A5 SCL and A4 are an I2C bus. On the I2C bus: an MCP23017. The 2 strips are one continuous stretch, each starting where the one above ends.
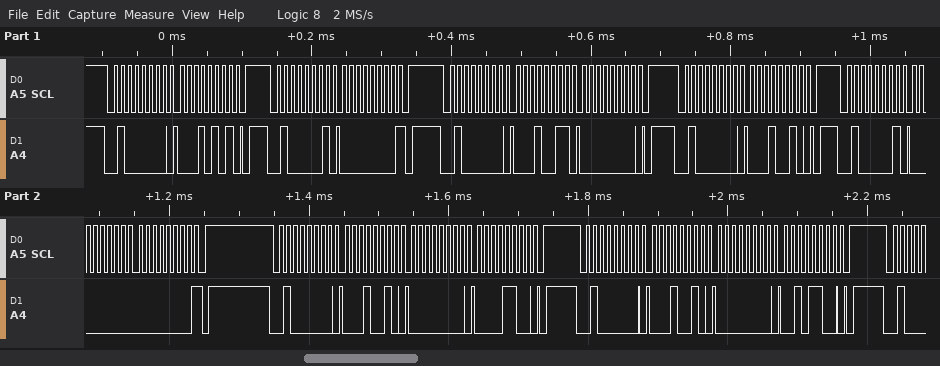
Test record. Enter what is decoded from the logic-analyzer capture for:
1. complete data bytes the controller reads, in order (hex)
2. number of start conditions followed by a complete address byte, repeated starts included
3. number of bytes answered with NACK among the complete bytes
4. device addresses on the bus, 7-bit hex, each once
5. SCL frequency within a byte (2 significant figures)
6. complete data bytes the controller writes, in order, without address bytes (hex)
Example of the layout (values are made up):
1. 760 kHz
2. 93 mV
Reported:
1. 00 00 00
2. 7
3. 2
4. 0x20
5. 100 kHz
6. 15 13 00 12 12 00 0C 12 00 2C
